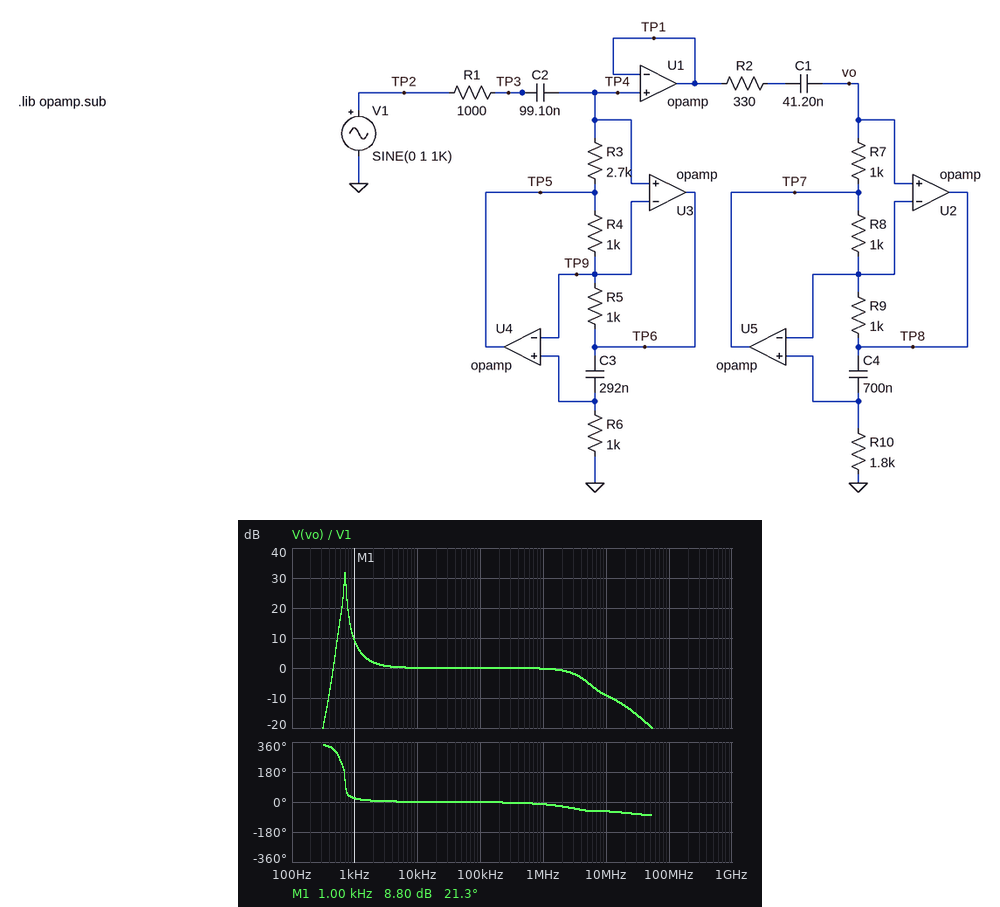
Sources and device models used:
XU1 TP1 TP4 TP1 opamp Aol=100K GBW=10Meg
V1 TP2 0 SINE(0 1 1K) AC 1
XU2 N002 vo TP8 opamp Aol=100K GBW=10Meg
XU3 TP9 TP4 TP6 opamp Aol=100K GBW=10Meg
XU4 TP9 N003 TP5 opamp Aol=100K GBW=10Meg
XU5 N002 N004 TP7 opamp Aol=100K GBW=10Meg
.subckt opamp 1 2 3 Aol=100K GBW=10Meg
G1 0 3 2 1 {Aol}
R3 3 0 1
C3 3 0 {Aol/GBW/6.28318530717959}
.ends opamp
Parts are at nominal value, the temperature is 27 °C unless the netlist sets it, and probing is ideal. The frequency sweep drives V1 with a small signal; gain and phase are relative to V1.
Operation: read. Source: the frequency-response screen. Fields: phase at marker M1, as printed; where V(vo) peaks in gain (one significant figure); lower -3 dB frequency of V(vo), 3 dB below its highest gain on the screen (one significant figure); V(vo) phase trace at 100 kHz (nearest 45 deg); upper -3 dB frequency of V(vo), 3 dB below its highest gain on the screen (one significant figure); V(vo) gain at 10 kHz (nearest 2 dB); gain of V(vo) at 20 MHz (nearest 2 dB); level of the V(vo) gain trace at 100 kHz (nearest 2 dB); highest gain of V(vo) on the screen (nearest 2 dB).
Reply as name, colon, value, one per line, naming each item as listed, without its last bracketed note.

phase at marker M1, as printed: 21.3 deg
where V(vo) peaks in gain: 700 Hz
lower -3 dB frequency of V(vo), 3 dB below its highest gain on the screen: 700 Hz
V(vo) phase trace at 100 kHz: 0 deg
upper -3 dB frequency of V(vo), 3 dB below its highest gain on the screen: 700 Hz
V(vo) gain at 10 kHz: 0 dB
gain of V(vo) at 20 MHz: -12 dB
level of the V(vo) gain trace at 100 kHz: 0 dB
highest gain of V(vo) on the screen: 32 dB
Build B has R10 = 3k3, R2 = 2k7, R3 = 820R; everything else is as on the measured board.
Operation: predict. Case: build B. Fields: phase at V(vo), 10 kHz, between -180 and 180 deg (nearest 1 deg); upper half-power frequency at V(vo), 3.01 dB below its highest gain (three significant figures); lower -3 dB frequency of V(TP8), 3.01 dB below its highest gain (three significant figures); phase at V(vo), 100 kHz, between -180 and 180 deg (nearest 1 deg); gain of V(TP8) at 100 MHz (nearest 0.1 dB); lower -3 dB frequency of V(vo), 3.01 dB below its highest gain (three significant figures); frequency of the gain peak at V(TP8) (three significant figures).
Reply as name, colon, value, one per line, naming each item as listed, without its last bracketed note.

phase at V(vo), 10 kHz, between -180 and 180 deg: 4 deg
upper half-power frequency at V(vo), 3.01 dB below its highest gain: 1.75 kHz
lower -3 dB frequency of V(TP8), 3.01 dB below its highest gain: 780 Hz
phase at V(vo), 100 kHz, between -180 and 180 deg: -5 deg
gain of V(TP8) at 100 MHz: -58.4 dB
lower -3 dB frequency of V(vo), 3.01 dB below its highest gain: 781 Hz
frequency of the gain peak at V(TP8): 1.09 kHz
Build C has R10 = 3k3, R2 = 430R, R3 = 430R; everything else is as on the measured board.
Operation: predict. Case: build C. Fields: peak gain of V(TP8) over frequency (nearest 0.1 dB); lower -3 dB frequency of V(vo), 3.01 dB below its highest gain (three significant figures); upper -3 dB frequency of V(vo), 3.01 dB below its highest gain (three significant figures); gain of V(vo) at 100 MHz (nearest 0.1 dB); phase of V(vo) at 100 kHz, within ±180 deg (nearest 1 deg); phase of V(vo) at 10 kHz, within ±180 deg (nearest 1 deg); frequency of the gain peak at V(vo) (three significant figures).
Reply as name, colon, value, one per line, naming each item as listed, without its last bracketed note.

peak gain of V(TP8) over frequency: 7.9 dB
lower -3 dB frequency of V(vo), 3.01 dB below its highest gain: 503 Hz
upper -3 dB frequency of V(vo), 3.01 dB below its highest gain: 534 Hz
gain of V(vo) at 100 MHz: -33.6 dB
phase of V(vo) at 100 kHz, within ±180 deg: -3 deg
phase of V(vo) at 10 kHz, within ±180 deg: 7 deg
frequency of the gain peak at V(vo): 517 Hz
